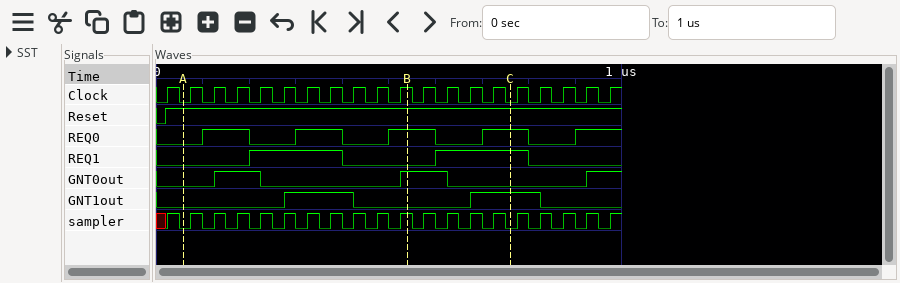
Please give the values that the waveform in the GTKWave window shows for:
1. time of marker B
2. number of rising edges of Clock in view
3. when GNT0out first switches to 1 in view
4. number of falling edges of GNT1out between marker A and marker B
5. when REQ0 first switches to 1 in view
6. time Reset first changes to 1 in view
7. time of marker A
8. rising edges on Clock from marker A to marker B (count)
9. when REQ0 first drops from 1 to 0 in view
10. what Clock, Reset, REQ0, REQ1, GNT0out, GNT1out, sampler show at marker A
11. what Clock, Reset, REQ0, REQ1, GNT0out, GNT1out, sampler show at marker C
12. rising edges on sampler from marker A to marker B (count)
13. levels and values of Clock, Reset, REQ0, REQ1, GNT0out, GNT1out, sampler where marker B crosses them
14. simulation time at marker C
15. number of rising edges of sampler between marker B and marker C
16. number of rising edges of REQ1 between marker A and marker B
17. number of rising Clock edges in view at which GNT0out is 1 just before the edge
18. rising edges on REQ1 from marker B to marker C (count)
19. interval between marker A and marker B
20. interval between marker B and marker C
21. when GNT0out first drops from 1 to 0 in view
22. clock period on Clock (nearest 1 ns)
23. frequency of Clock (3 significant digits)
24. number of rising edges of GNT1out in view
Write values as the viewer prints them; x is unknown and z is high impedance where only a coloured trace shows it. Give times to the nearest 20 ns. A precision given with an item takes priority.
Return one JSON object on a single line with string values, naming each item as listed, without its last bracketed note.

{"time of marker B": "540 ns", "number of rising edges of Clock in view": "20", "when GNT0out first switches to 1 in view": "120 ns", "number of falling edges of GNT1out between marker A and marker B": "1", "when REQ0 first switches to 1 in view": "100 ns", "time Reset first changes to 1 in view": "20 ns", "time of marker A": "60 ns", "rising edges on Clock from marker A to marker B": "10", "when REQ0 first drops from 1 to 0 in view": "200 ns", "what Clock, Reset, REQ0, REQ1, GNT0out, GNT1out, sampler show at marker A": "Clock=0, Reset=1, REQ0=0, REQ1=0, GNT0out=0, GNT1out=0, sampler=0", "what Clock, Reset, REQ0, REQ1, GNT0out, GNT1out, sampler show at marker C": "Clock=0, Reset=1, REQ0=1, REQ1=1, GNT0out=0, GNT1out=1, sampler=0", "rising edges on sampler from marker A to marker B": "10", "levels and values of Clock, Reset, REQ0, REQ1, GNT0out, GNT1out, sampler where marker B crosses them": "Clock=1, Reset=1, REQ0=1, REQ1=0, GNT0out=1, GNT1out=0, sampler=1", "simulation time at marker C": "760 ns", "number of rising edges of sampler between marker B and marker C": "4", "number of rising edges of REQ1 between marker A and marker B": "1", "number of rising Clock edges in view at which GNT0out is 1 just before the edge": "5", "rising edges on REQ1 from marker B to marker C": "1", "interval between marker A and marker B": "480 ns", "interval between marker B and marker C": "220 ns", "when GNT0out first drops from 1 to 0 in view": "220 ns", "clock period on Clock": "50 ns", "frequency of Clock": "20.0 MHz", "number of rising edges of GNT1out in view": "2"}
